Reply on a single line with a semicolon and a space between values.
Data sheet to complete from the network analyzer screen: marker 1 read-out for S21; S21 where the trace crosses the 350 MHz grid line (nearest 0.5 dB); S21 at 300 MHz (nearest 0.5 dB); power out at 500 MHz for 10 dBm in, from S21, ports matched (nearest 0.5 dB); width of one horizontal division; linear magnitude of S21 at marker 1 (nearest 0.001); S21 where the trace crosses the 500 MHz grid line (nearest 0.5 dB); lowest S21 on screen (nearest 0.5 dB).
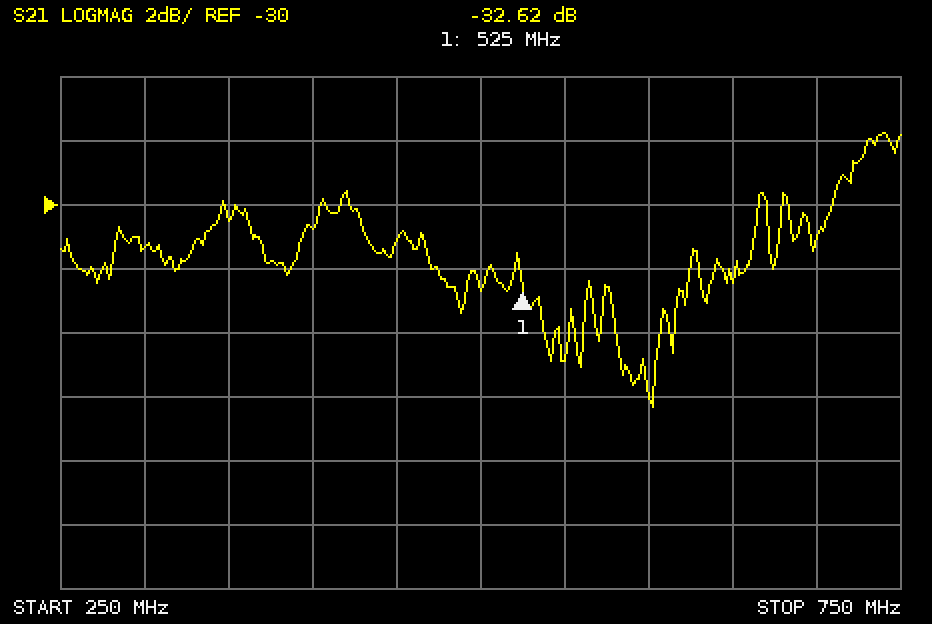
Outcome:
-32.62 dB; -30.5 dB; -31.5 dB; -22.5 dBm; 50 MHz; 0.023; -32.5 dB; -36.5 dB
